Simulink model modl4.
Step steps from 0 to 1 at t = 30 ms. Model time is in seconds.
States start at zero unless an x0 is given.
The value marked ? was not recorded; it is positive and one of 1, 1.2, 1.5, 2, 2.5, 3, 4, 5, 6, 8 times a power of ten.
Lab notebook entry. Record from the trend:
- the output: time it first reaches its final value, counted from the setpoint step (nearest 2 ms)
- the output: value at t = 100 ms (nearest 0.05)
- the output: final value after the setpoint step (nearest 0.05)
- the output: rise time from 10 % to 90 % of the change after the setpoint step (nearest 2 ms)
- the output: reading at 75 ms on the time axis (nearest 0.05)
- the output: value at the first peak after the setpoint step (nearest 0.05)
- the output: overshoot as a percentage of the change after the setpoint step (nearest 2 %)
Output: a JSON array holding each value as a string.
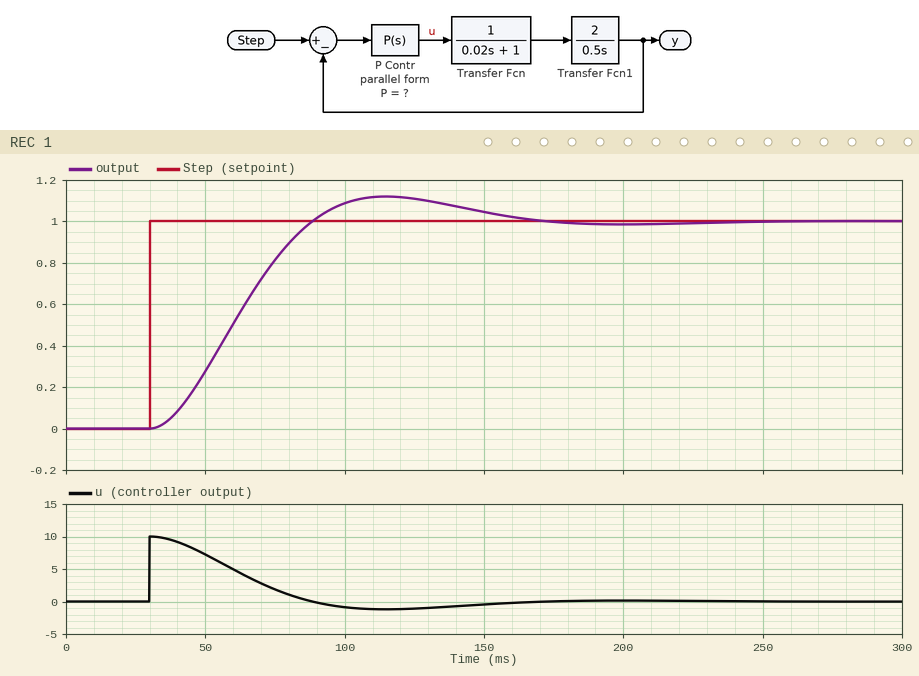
["58 ms", "1.10", "1.00", "40 ms", "0.80", "1.10", "12 %"]
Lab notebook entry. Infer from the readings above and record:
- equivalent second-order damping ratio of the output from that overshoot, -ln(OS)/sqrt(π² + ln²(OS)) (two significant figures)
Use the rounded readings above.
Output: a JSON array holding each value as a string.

["0.56"]
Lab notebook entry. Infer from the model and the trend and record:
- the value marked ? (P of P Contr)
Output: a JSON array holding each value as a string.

["10"]
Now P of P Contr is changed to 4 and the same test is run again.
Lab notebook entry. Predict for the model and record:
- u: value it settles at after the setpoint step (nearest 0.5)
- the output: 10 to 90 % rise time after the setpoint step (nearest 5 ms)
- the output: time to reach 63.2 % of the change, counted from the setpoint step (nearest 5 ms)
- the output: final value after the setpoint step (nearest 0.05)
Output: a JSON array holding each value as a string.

["0.0", "100 ms", "70 ms", "1.00"]
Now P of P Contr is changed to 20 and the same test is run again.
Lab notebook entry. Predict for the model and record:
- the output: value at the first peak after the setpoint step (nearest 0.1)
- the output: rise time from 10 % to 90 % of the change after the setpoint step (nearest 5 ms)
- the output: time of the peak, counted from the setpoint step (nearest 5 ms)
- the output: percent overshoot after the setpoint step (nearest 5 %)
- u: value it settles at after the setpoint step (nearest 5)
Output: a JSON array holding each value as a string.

["1.3", "25 ms", "55 ms", "25 %", "0"]
